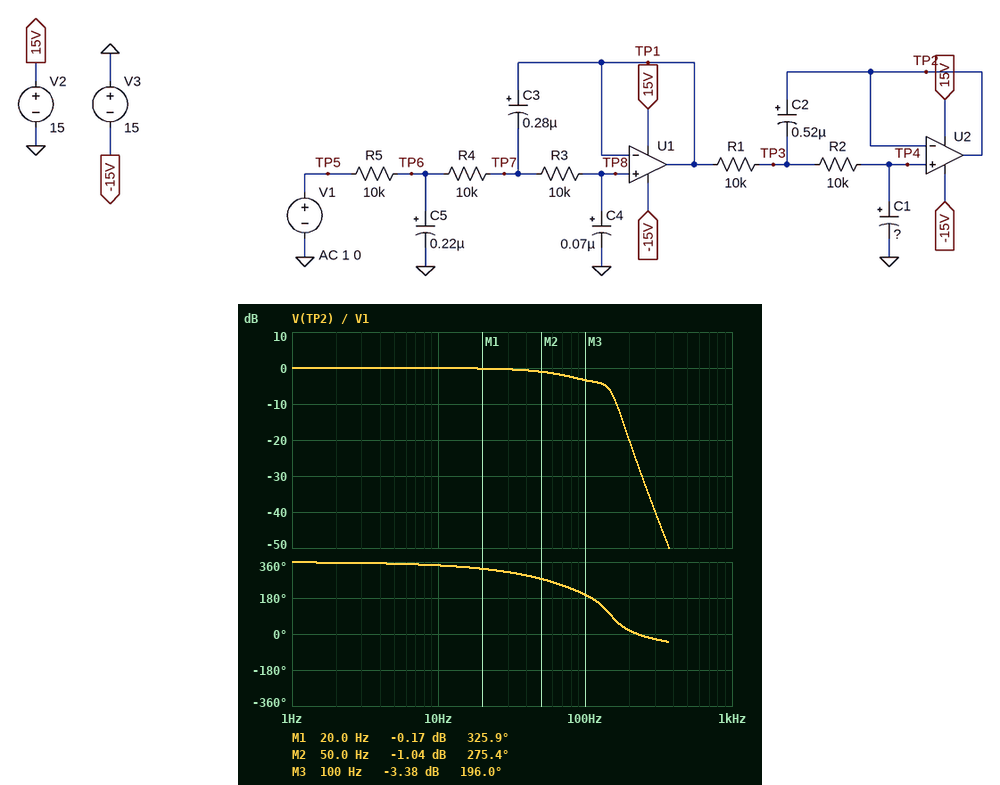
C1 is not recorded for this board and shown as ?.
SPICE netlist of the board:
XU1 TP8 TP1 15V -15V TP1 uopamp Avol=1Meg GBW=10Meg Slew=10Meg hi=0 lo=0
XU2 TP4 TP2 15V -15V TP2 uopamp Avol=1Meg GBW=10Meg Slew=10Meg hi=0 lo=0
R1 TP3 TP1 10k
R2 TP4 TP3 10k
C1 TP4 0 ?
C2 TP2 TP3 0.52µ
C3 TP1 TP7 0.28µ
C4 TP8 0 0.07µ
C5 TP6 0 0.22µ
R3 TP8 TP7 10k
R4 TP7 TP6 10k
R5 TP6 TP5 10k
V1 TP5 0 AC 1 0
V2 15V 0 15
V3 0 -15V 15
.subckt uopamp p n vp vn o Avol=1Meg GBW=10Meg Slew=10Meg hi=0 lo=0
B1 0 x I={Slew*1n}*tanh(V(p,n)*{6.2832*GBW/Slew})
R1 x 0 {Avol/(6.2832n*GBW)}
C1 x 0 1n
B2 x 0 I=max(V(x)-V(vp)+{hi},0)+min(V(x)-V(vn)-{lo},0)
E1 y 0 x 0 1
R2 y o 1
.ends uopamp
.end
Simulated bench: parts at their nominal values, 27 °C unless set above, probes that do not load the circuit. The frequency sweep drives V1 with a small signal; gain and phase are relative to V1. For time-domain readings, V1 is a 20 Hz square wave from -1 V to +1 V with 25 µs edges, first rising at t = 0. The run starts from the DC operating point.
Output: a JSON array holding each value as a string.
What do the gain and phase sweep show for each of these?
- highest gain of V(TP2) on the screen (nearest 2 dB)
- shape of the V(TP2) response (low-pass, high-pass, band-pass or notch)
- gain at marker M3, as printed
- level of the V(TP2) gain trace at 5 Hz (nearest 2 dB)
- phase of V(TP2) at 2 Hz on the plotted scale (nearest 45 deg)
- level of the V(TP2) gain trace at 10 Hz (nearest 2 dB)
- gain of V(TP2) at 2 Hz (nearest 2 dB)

["0 dB", "low-pass", "-3.38 dB", "0 dB", "360 deg", "0 dB", "0 dB"]
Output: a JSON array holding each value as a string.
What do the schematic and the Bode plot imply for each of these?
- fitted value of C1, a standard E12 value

["22 nF"]
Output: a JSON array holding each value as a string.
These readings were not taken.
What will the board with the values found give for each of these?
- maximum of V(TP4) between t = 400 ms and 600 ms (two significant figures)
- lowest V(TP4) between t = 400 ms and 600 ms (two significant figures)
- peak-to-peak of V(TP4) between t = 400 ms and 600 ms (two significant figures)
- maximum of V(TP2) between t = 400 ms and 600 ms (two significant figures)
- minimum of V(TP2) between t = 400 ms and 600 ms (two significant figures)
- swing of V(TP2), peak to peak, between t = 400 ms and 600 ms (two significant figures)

["1.0 V", "-1.0 V", "2.1 V", "1.0 V", "-1.0 V", "2.1 V"]
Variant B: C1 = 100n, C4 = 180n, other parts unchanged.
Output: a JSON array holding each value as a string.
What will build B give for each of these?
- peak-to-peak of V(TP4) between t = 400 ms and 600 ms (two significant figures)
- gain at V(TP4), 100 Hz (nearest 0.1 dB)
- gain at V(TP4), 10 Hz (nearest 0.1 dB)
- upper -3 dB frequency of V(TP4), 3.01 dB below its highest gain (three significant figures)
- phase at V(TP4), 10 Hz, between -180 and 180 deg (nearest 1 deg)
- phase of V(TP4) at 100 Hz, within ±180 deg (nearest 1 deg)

["2.0 V", "-20.5 dB", "-0.3 dB", "38.0 Hz", "-34 deg", "68 deg"]
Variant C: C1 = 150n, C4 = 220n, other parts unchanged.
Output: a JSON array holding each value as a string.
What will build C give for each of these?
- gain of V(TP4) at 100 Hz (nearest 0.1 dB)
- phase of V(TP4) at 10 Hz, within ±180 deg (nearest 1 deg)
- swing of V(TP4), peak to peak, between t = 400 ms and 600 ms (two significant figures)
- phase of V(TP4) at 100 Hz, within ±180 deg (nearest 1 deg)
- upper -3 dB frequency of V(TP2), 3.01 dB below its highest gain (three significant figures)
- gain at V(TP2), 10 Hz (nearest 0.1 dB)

["-27.0 dB", "-42 deg", "1.9 V", "58 deg", "28.7 Hz", "-0.4 dB"]
